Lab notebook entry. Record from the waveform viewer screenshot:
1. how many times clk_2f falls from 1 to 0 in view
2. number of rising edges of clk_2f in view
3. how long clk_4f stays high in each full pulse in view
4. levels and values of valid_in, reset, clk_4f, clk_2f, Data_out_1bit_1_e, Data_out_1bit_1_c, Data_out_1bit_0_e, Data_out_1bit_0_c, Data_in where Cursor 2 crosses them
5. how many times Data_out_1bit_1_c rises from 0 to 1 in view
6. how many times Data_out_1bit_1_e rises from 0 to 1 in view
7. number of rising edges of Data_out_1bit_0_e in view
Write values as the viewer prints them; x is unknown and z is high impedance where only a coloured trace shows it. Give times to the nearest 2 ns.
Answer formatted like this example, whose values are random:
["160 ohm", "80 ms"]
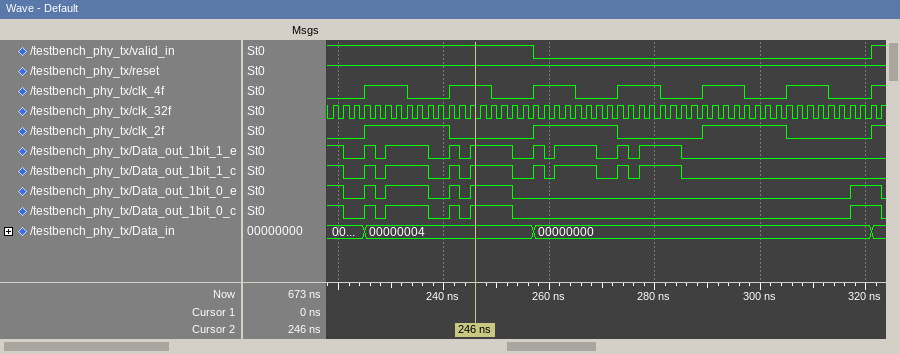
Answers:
["3", "4", "8 ns, 8 ns, 8 ns, 8 ns, 8 ns, 8 ns", "valid_in=1, reset=1, clk_4f=1, clk_2f=0, Data_out_1bit_1_e=1, Data_out_1bit_1_c=1, Data_out_1bit_0_e=1, Data_out_1bit_0_c=1, Data_in=00000004", "8", "8", "5"]
